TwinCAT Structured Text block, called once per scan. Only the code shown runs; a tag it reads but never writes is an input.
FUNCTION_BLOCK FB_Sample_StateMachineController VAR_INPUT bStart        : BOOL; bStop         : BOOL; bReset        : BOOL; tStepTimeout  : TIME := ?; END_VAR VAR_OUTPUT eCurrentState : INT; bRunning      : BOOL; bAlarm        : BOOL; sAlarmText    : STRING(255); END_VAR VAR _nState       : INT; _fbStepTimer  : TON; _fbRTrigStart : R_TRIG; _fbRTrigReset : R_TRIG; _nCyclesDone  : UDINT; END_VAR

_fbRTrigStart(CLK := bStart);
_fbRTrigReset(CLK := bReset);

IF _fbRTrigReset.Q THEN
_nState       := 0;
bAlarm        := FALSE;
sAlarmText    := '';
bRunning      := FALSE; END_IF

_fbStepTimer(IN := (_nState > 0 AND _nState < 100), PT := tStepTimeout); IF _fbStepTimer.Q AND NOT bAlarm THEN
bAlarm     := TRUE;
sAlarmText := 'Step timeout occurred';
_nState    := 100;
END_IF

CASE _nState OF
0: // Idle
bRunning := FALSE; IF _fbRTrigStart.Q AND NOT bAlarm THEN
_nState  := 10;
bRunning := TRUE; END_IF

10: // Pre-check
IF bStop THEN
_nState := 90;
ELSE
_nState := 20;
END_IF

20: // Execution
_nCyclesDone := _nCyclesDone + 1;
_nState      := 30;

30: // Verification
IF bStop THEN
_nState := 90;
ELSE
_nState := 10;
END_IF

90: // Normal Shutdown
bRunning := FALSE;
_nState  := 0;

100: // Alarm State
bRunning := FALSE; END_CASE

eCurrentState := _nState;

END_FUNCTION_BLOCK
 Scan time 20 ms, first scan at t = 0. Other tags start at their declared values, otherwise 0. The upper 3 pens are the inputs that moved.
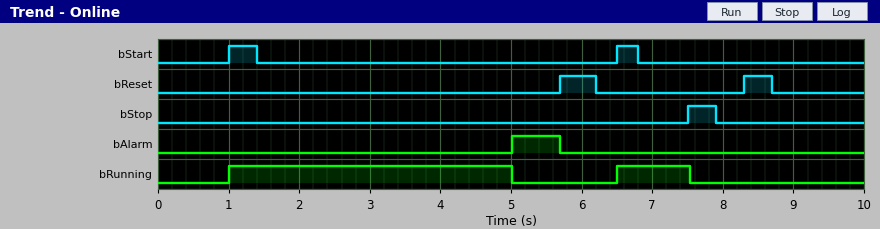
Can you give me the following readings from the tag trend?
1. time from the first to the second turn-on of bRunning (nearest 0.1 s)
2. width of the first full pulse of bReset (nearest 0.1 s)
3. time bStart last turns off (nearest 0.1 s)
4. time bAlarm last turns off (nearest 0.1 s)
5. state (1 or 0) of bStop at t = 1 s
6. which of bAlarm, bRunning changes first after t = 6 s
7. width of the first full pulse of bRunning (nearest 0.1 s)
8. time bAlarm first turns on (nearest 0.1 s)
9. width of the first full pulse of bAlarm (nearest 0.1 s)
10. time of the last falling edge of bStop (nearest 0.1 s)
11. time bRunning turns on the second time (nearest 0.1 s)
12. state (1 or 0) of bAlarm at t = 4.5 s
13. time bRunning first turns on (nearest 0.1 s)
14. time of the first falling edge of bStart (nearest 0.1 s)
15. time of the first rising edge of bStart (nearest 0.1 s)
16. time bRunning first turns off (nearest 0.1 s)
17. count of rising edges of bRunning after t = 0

5.5 s
0.5 s
6.8 s
5.7 s
0
bRunning
4.0 s
5.0 s
0.7 s
7.9 s
6.5 s
0
1.0 s
1.4 s
1.0 s
5.0 s
2
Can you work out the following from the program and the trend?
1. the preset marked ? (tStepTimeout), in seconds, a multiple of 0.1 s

4.0 s
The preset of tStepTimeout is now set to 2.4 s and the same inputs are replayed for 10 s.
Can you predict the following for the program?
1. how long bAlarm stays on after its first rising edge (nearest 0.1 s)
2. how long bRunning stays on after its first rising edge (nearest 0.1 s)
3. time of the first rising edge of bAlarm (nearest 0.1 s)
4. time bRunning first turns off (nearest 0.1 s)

2.3 s
2.4 s
3.4 s
3.4 s
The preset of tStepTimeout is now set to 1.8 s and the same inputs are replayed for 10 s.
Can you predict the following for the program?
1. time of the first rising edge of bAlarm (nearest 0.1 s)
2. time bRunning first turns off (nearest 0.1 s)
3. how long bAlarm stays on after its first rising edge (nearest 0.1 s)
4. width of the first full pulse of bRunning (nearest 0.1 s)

2.8 s
2.8 s
2.9 s
1.8 s
